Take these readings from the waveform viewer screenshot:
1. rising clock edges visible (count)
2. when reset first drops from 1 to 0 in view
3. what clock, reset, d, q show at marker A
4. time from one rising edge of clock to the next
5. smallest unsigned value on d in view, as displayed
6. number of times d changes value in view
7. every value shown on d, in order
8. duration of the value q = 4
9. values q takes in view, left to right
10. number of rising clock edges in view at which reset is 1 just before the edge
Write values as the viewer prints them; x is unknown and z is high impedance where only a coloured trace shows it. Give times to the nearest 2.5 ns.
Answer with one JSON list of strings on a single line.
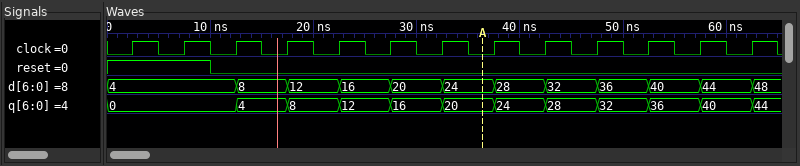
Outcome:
["13", "10 ns", "clock=0, reset=0, d=24, q=20", "5 ns", "4", "11", "4, 8, 12, 16, 20, 24, 28, 32, 36, 40, 44, 48", "5 ns", "0, 4, 8, 12, 16, 20, 24, 28, 32, 36, 40, 44", "2"]
